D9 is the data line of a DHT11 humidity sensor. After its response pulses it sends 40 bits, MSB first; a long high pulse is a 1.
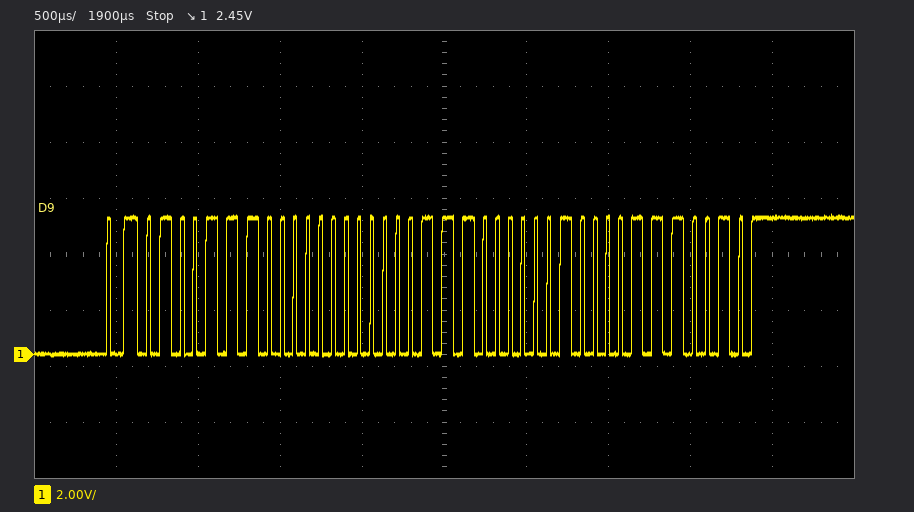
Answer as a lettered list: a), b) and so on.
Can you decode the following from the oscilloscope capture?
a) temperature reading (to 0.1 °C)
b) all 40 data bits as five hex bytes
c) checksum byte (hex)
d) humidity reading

a) 28.8 °C
b) 4E 00 1C 08 72
c) 0x72
d) 78 %
